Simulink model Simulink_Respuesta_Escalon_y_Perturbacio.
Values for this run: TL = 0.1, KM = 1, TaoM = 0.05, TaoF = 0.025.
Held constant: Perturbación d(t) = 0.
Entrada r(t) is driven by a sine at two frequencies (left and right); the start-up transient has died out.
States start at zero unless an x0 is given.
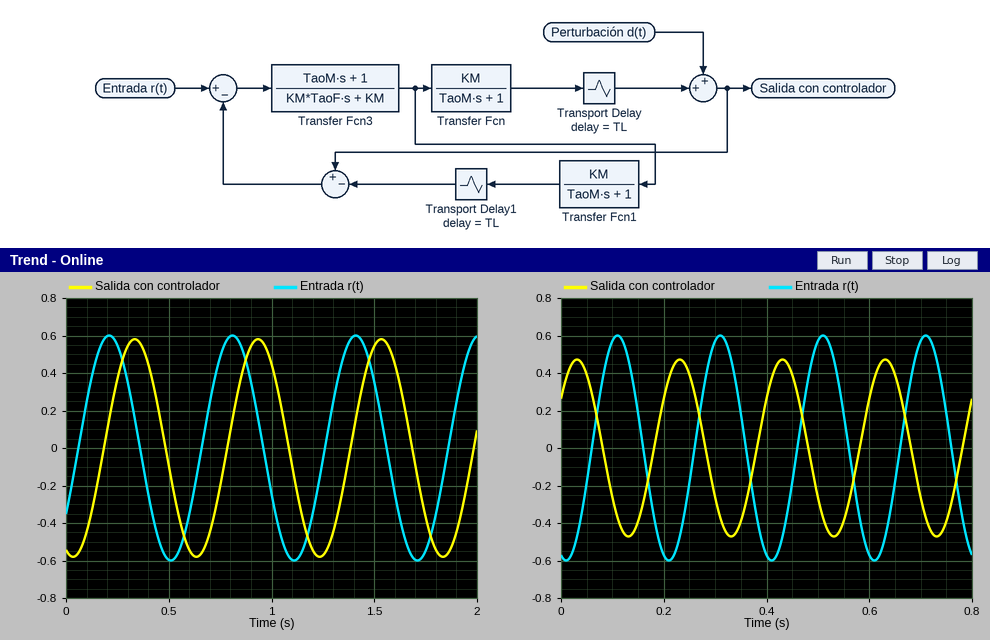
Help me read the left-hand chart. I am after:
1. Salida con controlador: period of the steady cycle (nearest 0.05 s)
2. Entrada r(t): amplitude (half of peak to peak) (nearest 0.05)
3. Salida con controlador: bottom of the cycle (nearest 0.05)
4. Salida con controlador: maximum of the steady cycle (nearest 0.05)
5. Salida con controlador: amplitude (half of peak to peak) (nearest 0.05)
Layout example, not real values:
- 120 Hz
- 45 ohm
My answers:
- 0.60 s
- 0.60
- -0.60
- 0.60
- 0.60
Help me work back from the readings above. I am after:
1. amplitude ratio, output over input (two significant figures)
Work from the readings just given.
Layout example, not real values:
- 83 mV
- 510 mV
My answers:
- 1.0
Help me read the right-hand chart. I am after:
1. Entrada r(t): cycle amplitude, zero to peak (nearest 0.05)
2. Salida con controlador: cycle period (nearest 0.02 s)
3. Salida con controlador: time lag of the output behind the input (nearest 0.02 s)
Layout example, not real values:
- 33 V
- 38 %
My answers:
- 0.60
- 0.20 s
- 0.12 s
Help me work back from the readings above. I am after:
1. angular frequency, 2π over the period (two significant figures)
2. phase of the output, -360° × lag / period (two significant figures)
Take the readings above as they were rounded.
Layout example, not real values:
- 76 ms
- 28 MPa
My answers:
- 31 rad/s
- -220°
